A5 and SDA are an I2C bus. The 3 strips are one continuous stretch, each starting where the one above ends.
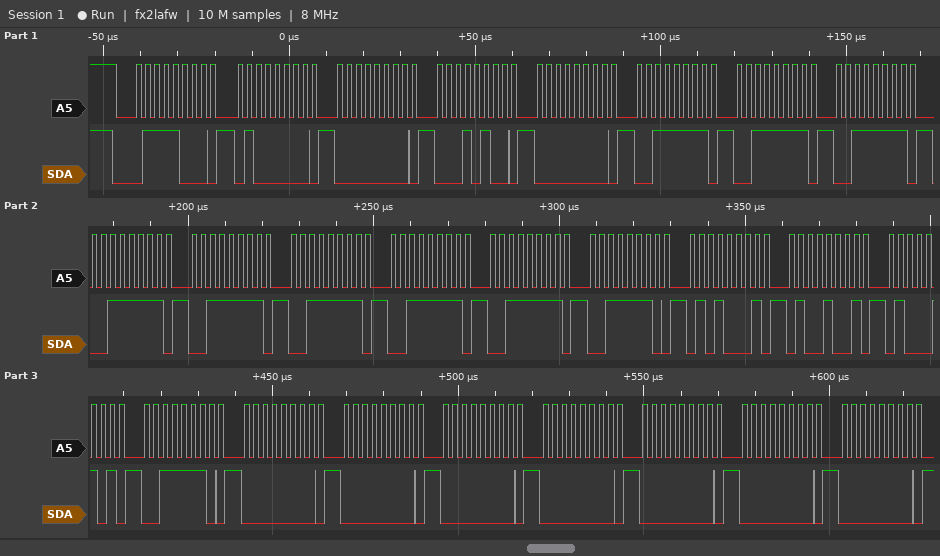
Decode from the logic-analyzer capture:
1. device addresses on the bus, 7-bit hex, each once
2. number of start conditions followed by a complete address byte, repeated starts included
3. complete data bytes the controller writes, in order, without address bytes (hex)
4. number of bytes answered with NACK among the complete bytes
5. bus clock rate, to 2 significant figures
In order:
0x3C
1
40 00 14 00 3F 3F 3F 3F 3F 3F 3F 3F 3E 51 49 45 3E 00 00 00 00 00 00 00
0
400 kHz
